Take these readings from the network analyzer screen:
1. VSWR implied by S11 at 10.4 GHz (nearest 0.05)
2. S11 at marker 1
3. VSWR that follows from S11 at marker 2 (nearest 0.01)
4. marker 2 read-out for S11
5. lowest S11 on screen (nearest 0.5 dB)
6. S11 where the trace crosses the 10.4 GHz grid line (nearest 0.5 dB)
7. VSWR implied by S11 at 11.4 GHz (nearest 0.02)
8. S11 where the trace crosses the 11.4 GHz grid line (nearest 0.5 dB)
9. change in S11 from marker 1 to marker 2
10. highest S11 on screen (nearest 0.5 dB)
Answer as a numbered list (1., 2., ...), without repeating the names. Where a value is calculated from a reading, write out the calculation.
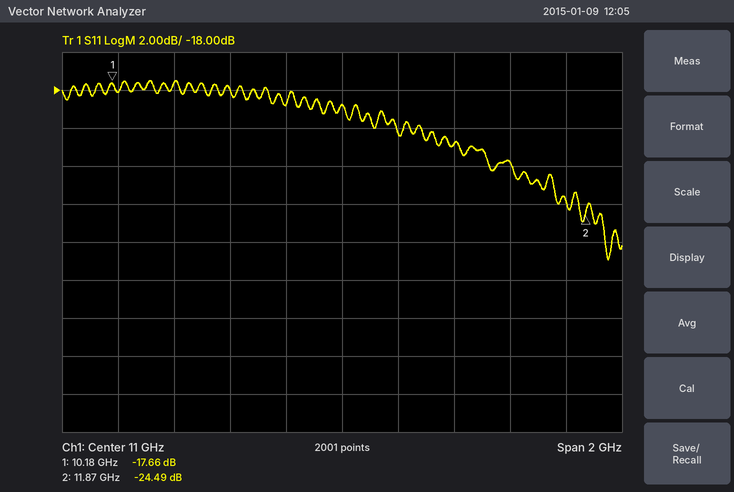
1. |Γ| = 10^(-17.5/20) = 0.1334; VSWR = (1 + 0.1334)/(1 − 0.1334) ≈ 1.31, so 1.30 to the nearest 0.05
2. -17.66 dB
3. (1 + 0.0596)/(1 − 0.0596) ≈ 1.13
4. -24.49 dB
5. -27.0 dB
6. -17.5 dB
7. |Γ| = 10^(-21/20) = 0.0891; VSWR = (1 + 0.0891)/(1 − 0.0891) ≈ 1.20
8. -21.0 dB
9. -24.49 − (-17.66) = -6.83 dB
10. -17.5 dB
